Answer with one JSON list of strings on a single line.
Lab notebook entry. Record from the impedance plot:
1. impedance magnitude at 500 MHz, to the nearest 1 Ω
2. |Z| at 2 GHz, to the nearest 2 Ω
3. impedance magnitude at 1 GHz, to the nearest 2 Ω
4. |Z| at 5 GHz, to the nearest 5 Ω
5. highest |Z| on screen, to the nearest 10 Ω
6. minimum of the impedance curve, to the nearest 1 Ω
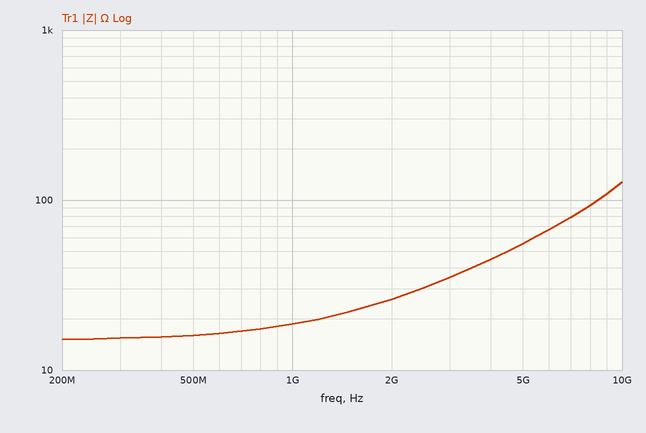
["16 Ω", "26 Ω", "18 Ω", "55 Ω", "130 Ω", "15 Ω"]
